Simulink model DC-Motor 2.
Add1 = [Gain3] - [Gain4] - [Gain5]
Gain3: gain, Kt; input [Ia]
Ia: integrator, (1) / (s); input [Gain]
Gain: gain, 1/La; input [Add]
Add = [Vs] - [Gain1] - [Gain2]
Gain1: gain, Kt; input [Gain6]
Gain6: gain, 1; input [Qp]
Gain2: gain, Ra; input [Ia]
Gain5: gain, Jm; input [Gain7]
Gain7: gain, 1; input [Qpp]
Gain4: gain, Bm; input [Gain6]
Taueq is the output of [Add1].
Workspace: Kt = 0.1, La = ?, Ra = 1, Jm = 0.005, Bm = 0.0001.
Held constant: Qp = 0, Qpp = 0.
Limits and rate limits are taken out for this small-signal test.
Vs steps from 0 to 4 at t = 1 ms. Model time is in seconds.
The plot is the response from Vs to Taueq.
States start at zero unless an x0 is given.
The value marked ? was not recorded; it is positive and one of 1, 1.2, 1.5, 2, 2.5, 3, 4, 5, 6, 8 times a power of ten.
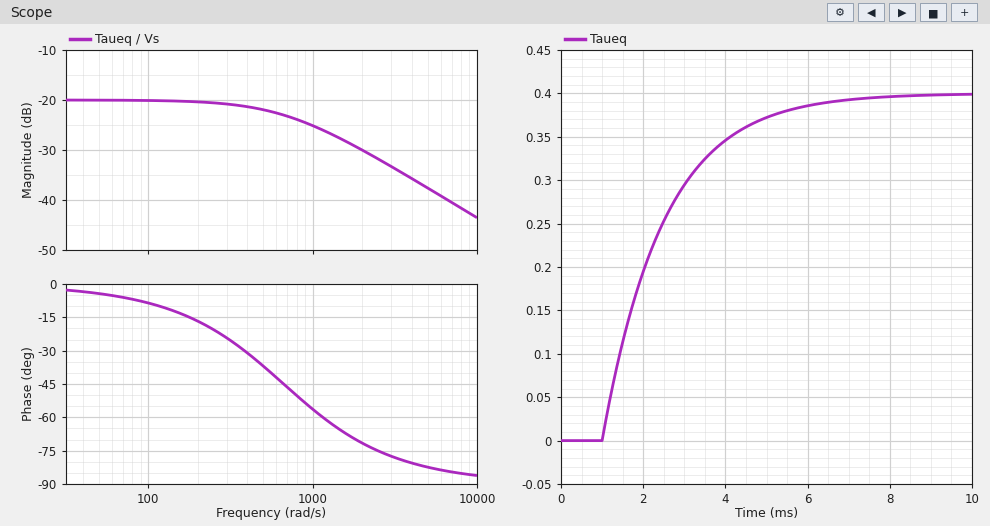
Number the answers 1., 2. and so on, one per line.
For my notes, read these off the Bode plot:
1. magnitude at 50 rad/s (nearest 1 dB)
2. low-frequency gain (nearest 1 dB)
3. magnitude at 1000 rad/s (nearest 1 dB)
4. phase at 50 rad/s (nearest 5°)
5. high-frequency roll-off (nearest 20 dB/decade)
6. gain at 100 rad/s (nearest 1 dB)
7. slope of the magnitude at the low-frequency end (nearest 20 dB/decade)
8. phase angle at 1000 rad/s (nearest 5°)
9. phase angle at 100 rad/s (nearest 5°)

1. -20 dB
2. -20 dB
3. -25 dB
4. -5°
5. -20 dB/decade
6. -20 dB
7. 0 dB/decade
8. -55°
9. -10°
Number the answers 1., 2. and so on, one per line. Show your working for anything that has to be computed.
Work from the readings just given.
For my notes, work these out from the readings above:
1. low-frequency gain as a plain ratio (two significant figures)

1. 10^(-20 / 20) = 0.10
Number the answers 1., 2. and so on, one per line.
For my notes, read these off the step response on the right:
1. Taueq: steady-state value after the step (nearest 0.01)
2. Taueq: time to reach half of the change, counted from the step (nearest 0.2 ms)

1. 0.40
2. 1.0 ms
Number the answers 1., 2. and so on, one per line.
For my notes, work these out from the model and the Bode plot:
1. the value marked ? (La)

1. 0.0015
